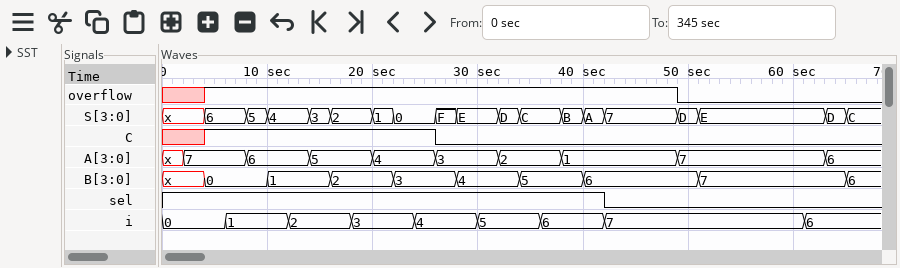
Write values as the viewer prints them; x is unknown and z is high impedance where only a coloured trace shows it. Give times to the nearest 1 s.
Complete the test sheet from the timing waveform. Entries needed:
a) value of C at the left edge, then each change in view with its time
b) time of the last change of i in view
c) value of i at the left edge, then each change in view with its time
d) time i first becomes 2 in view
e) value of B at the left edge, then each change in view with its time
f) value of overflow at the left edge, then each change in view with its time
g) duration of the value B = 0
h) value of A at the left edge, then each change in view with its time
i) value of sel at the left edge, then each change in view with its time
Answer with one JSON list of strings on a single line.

["x, 1 at 4 s, 0 at 26 s", "61 s", "0, 1 at 6 s, 2 at 12 s, 3 at 18 s, 4 at 24 s, 5 at 30 s, 6 at 36 s, 7 at 42 s, 6 at 61 s", "12 s", "x, 0 at 4 s, 1 at 10 s, 2 at 16 s, 3 at 22 s, 4 at 28 s, 5 at 34 s, 6 at 40 s, 7 at 51 s, 6 at 65 s", "x, 1 at 4 s, 0 at 49 s", "6 s", "x, 7 at 2 s, 6 at 8 s, 5 at 14 s, 4 at 20 s, 3 at 26 s, 2 at 32 s, 1 at 38 s, 7 at 49 s, 6 at 63 s", "1, 0 at 42 s"]
